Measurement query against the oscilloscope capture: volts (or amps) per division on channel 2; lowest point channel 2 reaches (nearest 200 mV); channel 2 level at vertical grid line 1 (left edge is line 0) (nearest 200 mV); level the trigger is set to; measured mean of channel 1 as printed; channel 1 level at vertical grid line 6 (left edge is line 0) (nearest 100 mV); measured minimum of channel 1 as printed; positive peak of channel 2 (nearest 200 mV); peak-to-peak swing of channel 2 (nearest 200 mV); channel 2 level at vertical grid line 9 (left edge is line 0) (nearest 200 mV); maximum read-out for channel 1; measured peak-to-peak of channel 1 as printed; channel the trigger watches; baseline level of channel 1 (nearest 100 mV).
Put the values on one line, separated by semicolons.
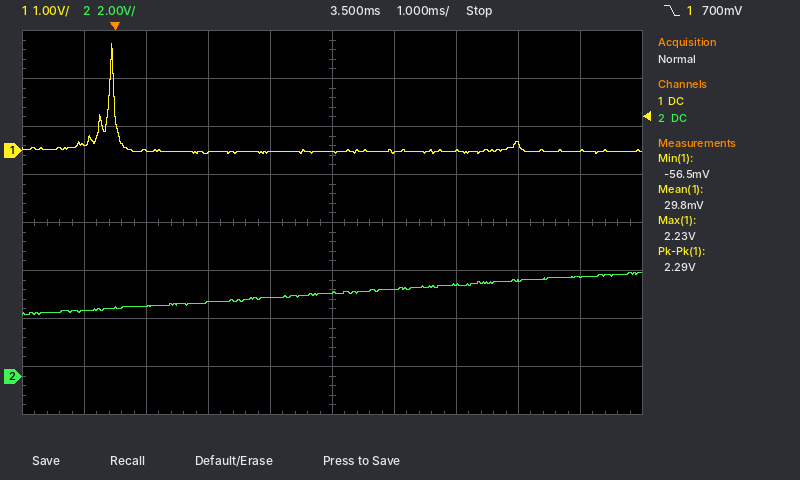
2 V; 2.6 V; 2.8 V; 700 mV; 29.8 mV; 0.0 V; -56.5 mV; 4.4 V; 1.8 V; 4.2 V; 2.23 V; 2.29 V; channel 1; 0.0 V
